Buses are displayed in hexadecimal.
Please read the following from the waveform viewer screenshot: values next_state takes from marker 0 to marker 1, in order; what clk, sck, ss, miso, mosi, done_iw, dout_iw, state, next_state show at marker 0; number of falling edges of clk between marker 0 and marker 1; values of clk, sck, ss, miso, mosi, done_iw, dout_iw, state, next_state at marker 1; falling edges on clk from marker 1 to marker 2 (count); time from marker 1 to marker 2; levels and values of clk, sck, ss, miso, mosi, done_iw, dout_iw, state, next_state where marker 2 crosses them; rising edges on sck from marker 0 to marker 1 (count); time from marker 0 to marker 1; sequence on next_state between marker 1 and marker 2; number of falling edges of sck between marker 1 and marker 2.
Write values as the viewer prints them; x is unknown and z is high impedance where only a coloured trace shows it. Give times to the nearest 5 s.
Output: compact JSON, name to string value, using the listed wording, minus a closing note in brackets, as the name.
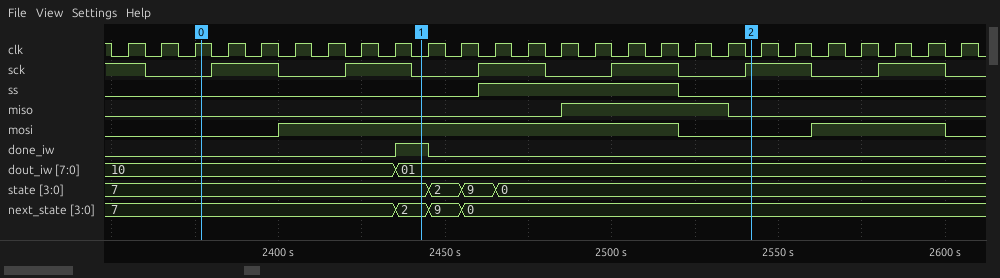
{"values next_state takes from marker 0 to marker 1, in order": "7, 2", "what clk, sck, ss, miso, mosi, done_iw, dout_iw, state, next_state show at marker 0": "clk=1, sck=0, ss=0, miso=0, mosi=0, done_iw=0, dout_iw=10, state=7, next_state=7", "number of falling edges of clk between marker 0 and marker 1": "7", "values of clk, sck, ss, miso, mosi, done_iw, dout_iw, state, next_state at marker 1": "clk=0, sck=0, ss=0, miso=0, mosi=1, done_iw=1, dout_iw=01, state=7, next_state=2", "falling edges on clk from marker 1 to marker 2": "10", "time from marker 1 to marker 2": "100 s", "levels and values of clk, sck, ss, miso, mosi, done_iw, dout_iw, state, next_state where marker 2 crosses them": "clk=0, sck=1, ss=0, miso=0, mosi=0, done_iw=0, dout_iw=01, state=0, next_state=0", "rising edges on sck from marker 0 to marker 1": "2", "time from marker 0 to marker 1": "65 s", "sequence on next_state between marker 1 and marker 2": "2, 9, 0", "number of falling edges of sck between marker 1 and marker 2": "2"}
